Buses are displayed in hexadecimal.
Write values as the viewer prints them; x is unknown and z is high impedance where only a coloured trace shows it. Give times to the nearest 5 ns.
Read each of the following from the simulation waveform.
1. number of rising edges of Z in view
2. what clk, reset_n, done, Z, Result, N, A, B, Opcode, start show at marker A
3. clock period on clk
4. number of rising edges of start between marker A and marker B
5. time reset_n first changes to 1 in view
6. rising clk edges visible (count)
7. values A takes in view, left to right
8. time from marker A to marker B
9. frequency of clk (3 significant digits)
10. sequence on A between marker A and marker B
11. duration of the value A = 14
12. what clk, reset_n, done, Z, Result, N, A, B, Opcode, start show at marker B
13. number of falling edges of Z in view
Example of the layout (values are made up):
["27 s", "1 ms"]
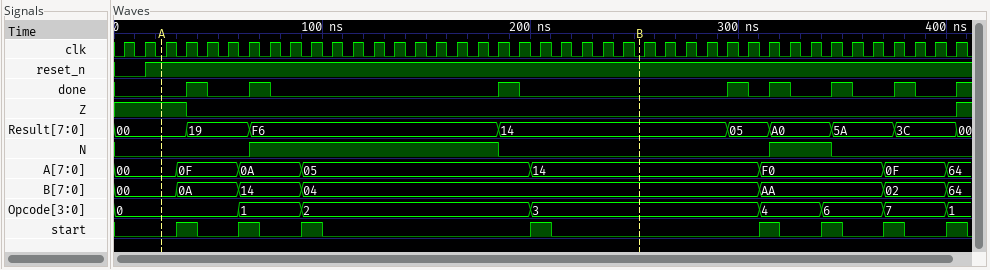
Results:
["1", "clk=0, reset_n=1, done=0, Z=1, Result=00, N=0, A=00, B=00, Opcode=0, start=0", "10 ns", "4", "15 ns", "41", "00, 0F, 0A, 05, 14, F0, 0F, 64", "230 ns", "100 MHz", "00, 0F, 0A, 05, 14", "110 ns", "clk=0, reset_n=1, done=0, Z=0, Result=14, N=0, A=14, B=04, Opcode=3, start=0", "1"]
